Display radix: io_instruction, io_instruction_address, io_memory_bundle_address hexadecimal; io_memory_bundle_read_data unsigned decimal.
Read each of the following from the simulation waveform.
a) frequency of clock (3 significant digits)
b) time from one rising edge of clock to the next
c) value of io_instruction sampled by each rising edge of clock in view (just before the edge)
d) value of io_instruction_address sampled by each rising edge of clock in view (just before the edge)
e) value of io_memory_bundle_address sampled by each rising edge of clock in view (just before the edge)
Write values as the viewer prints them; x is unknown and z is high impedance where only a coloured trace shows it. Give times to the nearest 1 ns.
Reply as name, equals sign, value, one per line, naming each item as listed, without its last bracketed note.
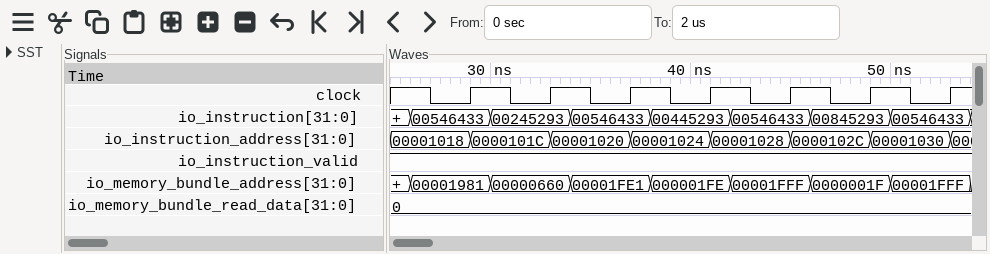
frequency of clock = 250 MHz
time from one rising edge of clock to the next = 4 ns
value of io_instruction sampled by each rising edge of clock in view = 00546433, 00245293, 00546433, 00445293, 00546433, 00845293, 00546433
value of io_instruction_address sampled by each rising edge of clock in view = 00001018, 0000101C, 00001020, 00001024, 00001028, 0000102C, 00001030
value of io_memory_bundle_address sampled by each rising edge of clock in view = 00001981, 00000660, 00001FE1, 000001FE, 00001FFF, 0000001F, 00001FFF
